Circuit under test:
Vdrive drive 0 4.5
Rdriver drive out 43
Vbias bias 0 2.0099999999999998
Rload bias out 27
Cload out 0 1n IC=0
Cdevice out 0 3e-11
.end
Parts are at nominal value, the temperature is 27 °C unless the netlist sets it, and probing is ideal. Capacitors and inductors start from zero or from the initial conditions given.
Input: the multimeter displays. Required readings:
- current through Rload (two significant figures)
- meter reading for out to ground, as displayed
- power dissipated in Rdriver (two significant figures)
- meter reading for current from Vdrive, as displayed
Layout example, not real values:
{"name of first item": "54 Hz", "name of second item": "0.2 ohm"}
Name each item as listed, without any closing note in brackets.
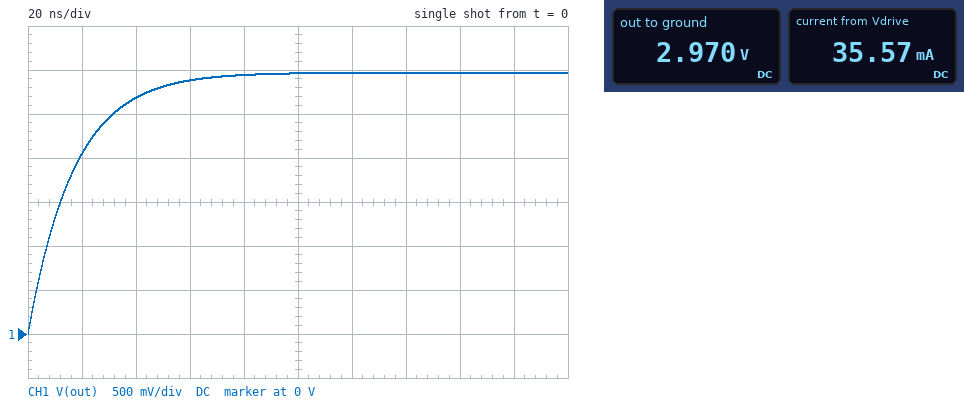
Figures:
{"current through Rload": "36 mA", "meter reading for out to ground, as displayed": "2.970 V", "power dissipated in Rdriver": "54 mW", "meter reading for current from Vdrive, as displayed": "35.57 mA"}
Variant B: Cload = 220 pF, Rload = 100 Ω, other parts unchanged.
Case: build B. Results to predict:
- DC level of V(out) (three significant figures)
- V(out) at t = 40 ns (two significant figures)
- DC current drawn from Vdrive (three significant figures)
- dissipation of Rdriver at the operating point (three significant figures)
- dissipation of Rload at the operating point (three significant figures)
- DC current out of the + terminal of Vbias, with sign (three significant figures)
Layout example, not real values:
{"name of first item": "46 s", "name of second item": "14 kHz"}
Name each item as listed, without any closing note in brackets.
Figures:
{"DC level of V(out)": "3.75 V", "V(out) at t = 40 ns": "3.7 V", "DC current drawn from Vdrive": "17.4 mA", "dissipation of Rdriver at the operating point": "13.0 mW", "dissipation of Rload at the operating point": "30.3 mW", "DC current out of the + terminal of Vbias, with sign": "-17.4 mA"}
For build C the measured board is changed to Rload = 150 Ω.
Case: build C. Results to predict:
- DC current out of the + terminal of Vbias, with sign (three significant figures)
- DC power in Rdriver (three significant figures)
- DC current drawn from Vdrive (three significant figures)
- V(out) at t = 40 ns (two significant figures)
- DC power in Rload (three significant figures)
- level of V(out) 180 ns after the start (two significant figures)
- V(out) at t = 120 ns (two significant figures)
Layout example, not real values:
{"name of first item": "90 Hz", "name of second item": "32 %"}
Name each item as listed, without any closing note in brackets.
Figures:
{"DC current out of the + terminal of Vbias, with sign": "-12.9 mA", "DC power in Rdriver": "7.16 mW", "DC current drawn from Vdrive": "12.9 mA", "V(out) at t = 40 ns": "2.7 V", "DC power in Rload": "25.0 mW", "level of V(out) 180 ns after the start": "3.9 V", "V(out) at t = 120 ns": "3.8 V"}
